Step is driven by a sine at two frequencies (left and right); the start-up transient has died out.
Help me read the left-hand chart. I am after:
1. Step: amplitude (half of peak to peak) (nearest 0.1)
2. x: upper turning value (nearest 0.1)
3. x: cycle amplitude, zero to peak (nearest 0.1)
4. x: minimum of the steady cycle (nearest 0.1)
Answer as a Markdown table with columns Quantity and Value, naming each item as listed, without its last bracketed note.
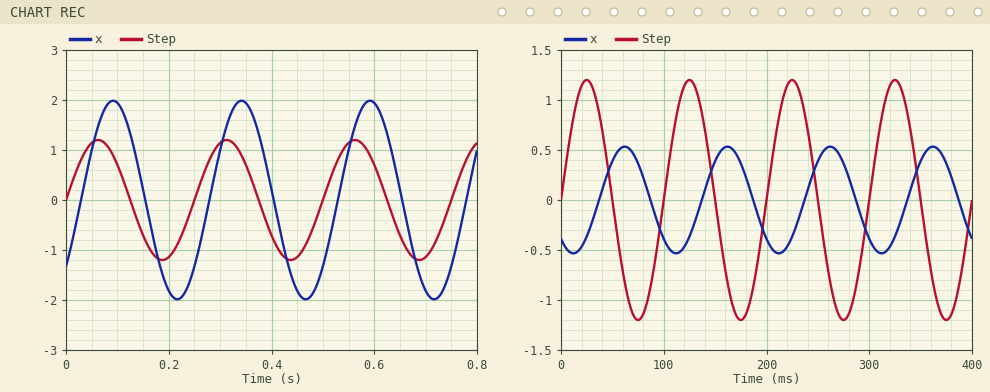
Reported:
| Quantity | Value |
|---|---|
| Step: amplitude (half of peak to peak) | 1.2 |
| x: upper turning value | 2.0 |
| x: cycle amplitude, zero to peak | 2.0 |
| x: minimum of the steady cycle | -2.0 |
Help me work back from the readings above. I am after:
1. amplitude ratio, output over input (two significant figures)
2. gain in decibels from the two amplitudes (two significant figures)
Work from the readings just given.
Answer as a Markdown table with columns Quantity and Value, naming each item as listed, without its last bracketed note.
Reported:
| Quantity | Value |
|---|---|
| amplitude ratio, output over input | 1.7 |
| gain in decibels from the two amplitudes | 4.4 dB |
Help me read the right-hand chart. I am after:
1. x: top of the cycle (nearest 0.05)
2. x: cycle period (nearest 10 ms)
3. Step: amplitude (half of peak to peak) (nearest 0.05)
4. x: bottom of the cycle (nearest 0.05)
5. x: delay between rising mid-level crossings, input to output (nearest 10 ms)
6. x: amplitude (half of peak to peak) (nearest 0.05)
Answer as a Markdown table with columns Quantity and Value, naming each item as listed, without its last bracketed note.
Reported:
| Quantity | Value |
|---|---|
| x: top of the cycle | 0.55 |
| x: cycle period | 100 ms |
| Step: amplitude (half of peak to peak) | 1.20 |
| x: bottom of the cycle | -0.55 |
| x: delay between rising mid-level crossings, input to output | 40 ms |
| x: amplitude (half of peak to peak) | 0.55 |
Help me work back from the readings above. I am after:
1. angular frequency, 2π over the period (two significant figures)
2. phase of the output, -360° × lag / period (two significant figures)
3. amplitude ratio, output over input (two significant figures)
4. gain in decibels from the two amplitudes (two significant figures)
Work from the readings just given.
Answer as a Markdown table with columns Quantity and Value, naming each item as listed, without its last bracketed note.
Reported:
| Quantity | Value |
|---|---|
| angular frequency, 2π over the period | 0.063 rad/ms |
| phase of the output, -360° × lag / period | -140° |
| amplitude ratio, output over input | 0.46 |
| gain in decibels from the two amplitudes | -6.8 dB |
